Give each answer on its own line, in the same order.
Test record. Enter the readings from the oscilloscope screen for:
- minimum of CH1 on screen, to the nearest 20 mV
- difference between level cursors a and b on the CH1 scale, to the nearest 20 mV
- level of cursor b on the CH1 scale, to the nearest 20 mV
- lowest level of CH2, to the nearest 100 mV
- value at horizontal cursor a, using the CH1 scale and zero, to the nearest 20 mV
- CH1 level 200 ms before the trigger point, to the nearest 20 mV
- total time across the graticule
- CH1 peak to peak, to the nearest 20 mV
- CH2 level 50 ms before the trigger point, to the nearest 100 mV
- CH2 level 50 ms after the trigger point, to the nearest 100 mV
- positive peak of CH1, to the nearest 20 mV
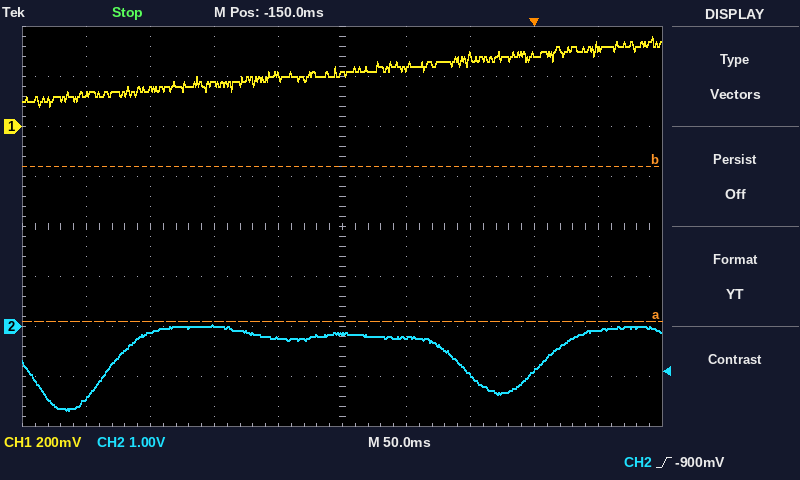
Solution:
80 mV
620 mV
-160 mV
-1.7 V
-780 mV
200 mV
500 ms
280 mV
-1.0 V
-100 mV
360 mV
